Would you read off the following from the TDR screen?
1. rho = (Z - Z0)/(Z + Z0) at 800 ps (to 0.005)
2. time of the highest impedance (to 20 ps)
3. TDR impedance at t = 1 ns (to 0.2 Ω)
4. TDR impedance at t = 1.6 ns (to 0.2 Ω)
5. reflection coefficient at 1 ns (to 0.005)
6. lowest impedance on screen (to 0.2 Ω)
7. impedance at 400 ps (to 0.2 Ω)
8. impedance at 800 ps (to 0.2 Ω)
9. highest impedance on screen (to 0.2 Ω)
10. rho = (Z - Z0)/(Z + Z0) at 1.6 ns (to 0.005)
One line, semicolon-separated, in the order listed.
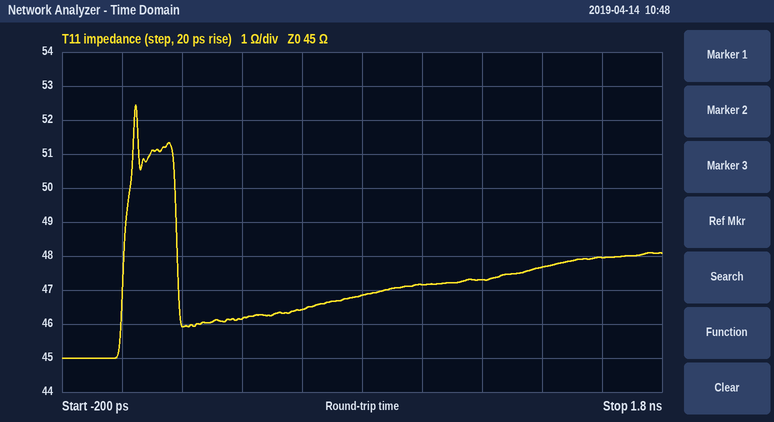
+0.020; 40 ps; 47.2 Ω; 48.0 Ω; +0.025; 45.0 Ω; 46.2 Ω; 46.8 Ω; 52.4 Ω; +0.030
